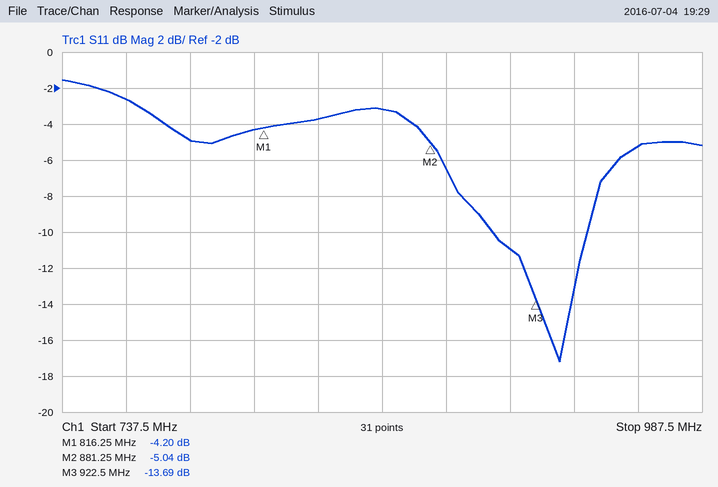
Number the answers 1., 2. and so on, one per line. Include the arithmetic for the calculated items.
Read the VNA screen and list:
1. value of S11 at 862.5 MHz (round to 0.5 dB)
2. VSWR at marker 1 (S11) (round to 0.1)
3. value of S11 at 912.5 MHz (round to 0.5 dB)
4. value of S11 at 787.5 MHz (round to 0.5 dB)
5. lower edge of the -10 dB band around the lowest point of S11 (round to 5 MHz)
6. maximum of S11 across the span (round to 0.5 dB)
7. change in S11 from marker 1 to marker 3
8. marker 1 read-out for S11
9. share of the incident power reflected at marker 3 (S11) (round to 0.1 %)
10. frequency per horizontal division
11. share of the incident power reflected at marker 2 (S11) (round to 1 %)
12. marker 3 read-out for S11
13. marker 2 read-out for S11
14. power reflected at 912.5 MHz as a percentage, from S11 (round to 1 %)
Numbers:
1. -3.0 dB
2. (1 + 0.6166)/(1 − 0.6166) ≈ 4.2
3. -11.0 dB
4. -5.0 dB
5. 905 MHz
6. -1.5 dB
7. -13.69 − (-4.2) = -9.49 dB
8. -4.20 dB
9. 10^(-13.69/10) ≈ 4.3 %
10. 25 MHz
11. 10^(-5.04/10) ≈ 31 %
12. -13.69 dB
13. -5.04 dB
14. 10^(-11/10) ≈ 8 %
